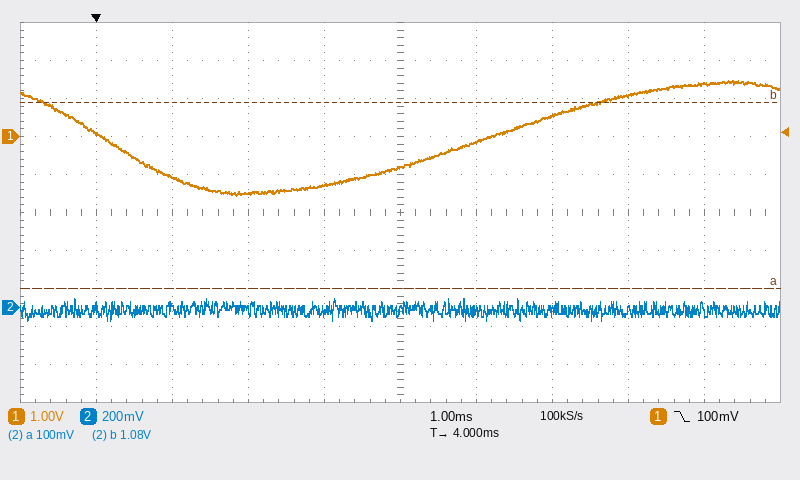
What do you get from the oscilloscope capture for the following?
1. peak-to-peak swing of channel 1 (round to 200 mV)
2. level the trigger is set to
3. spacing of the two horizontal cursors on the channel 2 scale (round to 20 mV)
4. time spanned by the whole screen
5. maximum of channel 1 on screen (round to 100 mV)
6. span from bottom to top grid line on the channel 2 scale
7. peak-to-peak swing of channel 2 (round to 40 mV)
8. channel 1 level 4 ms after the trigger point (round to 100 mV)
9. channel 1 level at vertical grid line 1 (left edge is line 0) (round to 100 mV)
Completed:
3.0 V
100 mV
980 mV
10 ms
1.5 V
2 V
120 mV
-800 mV
100 mV
